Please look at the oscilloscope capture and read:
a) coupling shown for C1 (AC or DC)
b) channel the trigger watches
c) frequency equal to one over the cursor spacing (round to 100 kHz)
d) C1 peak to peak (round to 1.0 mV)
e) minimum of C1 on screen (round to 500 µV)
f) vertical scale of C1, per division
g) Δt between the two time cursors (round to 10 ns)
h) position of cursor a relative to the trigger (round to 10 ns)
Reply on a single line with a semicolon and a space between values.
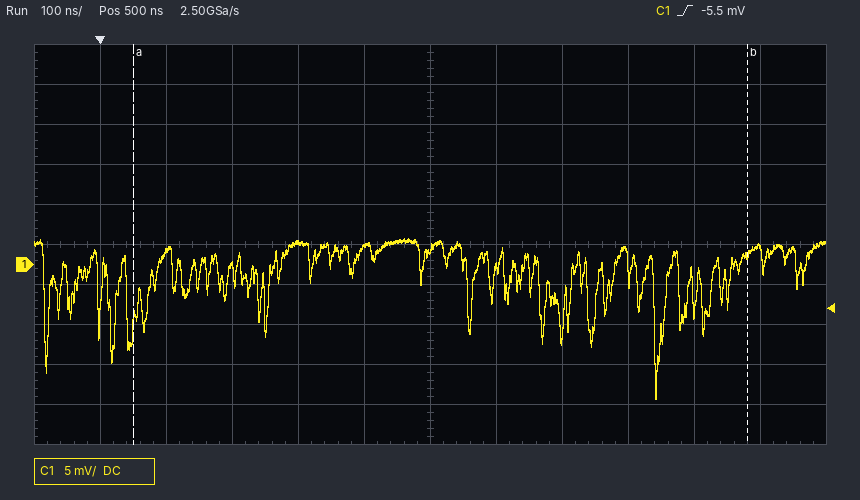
DC; C1; 1.1 MHz; 20.0 mV; -17.0 mV; 5 mV; 930 ns; +50 ns
